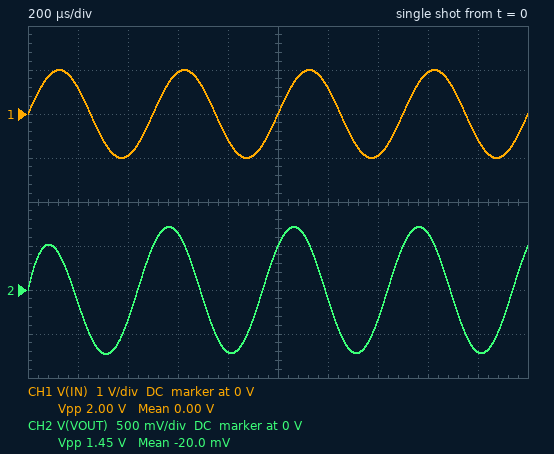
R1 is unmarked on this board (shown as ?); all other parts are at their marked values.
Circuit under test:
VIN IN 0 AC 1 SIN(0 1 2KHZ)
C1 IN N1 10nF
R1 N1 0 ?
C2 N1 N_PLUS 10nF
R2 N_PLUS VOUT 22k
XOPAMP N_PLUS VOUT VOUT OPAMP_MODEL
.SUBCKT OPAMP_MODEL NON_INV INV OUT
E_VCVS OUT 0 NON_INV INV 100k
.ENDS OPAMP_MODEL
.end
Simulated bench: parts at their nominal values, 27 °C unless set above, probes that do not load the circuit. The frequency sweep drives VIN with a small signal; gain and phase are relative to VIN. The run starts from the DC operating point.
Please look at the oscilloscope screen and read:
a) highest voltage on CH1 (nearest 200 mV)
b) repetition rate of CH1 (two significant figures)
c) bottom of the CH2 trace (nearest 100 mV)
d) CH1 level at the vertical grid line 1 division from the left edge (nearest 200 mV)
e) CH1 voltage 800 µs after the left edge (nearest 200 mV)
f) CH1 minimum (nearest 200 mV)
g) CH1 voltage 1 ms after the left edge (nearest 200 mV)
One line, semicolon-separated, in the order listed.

1.0 V; 2.0 kHz; -700 mV; 600 mV; -600 mV; -1.0 V; 0 V
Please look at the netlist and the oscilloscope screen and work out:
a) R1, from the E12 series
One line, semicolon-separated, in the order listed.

8.2 kΩ
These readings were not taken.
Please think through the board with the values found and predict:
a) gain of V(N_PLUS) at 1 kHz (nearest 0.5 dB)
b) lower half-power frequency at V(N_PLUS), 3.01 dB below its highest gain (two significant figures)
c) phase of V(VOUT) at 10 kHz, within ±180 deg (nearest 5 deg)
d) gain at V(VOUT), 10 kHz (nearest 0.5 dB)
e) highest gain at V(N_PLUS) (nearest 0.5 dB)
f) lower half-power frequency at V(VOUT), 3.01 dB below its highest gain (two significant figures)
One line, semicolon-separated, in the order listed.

-7.0 dB; 1.9 kHz; 10 deg; 0 dB; 0 dB; 1.9 kHz
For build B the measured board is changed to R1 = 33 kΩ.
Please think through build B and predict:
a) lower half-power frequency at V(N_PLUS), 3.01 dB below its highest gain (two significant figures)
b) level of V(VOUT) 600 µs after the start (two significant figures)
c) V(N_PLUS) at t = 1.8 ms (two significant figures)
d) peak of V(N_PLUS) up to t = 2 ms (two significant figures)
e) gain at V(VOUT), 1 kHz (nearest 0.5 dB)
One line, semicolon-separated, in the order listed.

480 Hz; 930 mV; -740 mV; 970 mV; -1.0 dB
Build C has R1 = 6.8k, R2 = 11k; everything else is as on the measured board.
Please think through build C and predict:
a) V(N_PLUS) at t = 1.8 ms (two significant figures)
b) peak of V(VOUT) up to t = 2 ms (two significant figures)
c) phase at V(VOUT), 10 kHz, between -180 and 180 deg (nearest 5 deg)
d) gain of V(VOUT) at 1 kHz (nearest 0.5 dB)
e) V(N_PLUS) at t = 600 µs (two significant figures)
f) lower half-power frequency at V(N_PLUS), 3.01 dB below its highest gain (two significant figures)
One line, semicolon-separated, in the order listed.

-650 mV; 650 mV; 15 deg; -8.0 dB; 550 mV; 2.3 kHz
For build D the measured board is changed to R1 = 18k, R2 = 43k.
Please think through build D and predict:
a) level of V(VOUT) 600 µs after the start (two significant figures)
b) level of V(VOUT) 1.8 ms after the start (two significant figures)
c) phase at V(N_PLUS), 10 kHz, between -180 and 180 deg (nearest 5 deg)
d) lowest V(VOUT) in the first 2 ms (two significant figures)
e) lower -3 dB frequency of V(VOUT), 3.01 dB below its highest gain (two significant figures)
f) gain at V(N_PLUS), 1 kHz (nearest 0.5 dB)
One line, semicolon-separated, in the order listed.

900 mV; -790 mV; 5 deg; -970 mV; 880 Hz; -2.5 dB
